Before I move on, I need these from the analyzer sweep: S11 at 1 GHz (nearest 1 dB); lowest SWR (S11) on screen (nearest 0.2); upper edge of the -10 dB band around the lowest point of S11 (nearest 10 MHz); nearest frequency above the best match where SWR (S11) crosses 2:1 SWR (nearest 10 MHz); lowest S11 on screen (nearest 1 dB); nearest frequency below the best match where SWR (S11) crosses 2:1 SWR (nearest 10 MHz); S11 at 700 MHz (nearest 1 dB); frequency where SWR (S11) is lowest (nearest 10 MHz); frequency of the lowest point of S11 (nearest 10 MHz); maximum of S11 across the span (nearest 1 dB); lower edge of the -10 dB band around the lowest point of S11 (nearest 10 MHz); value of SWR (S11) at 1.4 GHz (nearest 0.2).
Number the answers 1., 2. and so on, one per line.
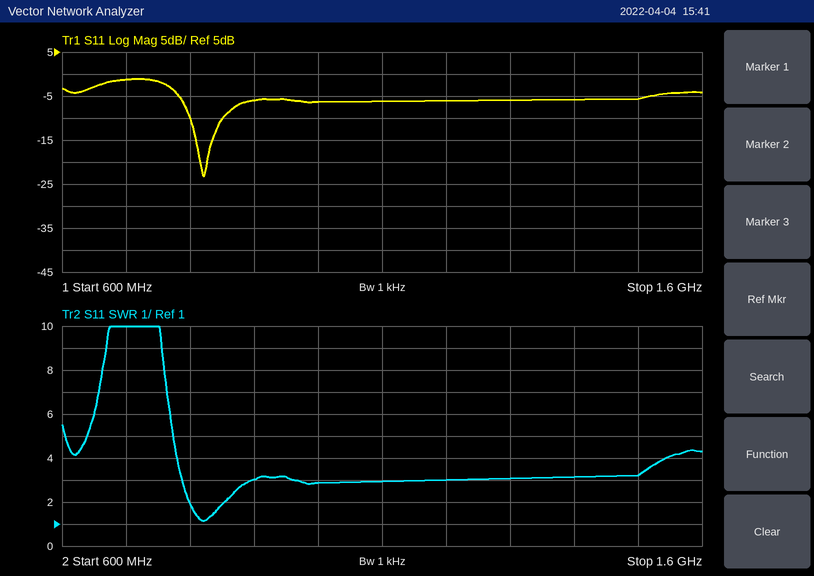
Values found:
1. -6 dB
2. 1.2
3. 850 MHz
4. 850 MHz
5. -23 dB
6. 800 MHz
7. -1 dB
8. 820 MHz
9. 820 MHz
10. -1 dB
11. 800 MHz
12. 3.2
